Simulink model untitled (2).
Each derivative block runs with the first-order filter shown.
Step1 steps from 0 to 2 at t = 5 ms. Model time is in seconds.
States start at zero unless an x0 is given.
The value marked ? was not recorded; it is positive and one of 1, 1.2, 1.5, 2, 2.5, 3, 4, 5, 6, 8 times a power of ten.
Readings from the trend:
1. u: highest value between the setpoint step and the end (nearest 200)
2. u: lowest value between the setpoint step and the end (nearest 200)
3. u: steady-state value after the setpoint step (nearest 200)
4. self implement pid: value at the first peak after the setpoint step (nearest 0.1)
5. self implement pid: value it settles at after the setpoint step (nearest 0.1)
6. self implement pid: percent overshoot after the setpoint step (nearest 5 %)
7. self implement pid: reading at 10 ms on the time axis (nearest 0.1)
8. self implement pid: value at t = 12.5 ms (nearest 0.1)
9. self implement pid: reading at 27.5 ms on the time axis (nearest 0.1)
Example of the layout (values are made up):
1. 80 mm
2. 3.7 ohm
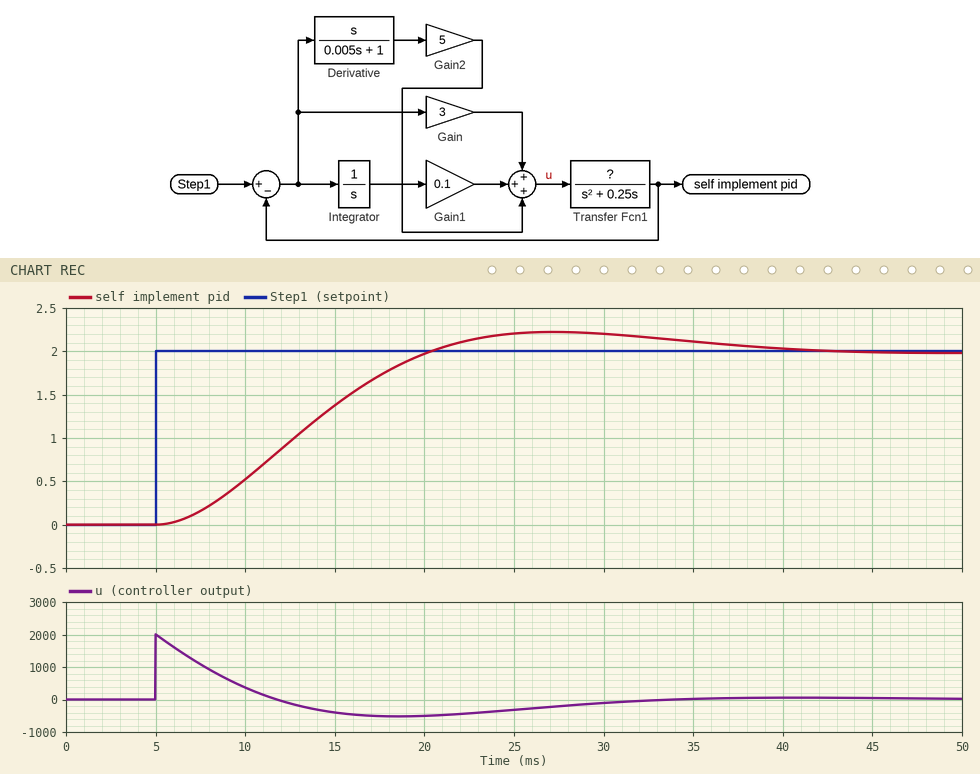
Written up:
1. 2000
2. -600
3. 0
4. 2.2
5. 2.0
6. 10 %
7. 0.5
8. 1.0
9. 2.2
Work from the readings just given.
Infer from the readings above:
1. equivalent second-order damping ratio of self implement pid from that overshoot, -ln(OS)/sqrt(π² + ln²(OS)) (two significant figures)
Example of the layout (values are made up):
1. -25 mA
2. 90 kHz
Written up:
1. 0.59
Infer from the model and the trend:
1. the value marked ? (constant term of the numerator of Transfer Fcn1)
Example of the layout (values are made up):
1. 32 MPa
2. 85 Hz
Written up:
1. 30
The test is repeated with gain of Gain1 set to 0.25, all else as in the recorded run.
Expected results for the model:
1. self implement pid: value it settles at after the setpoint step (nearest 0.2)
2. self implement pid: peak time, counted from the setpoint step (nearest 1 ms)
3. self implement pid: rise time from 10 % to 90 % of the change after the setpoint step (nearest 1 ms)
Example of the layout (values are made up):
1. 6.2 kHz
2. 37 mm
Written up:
1. 2.0
2. 22 ms
3. 10 ms
